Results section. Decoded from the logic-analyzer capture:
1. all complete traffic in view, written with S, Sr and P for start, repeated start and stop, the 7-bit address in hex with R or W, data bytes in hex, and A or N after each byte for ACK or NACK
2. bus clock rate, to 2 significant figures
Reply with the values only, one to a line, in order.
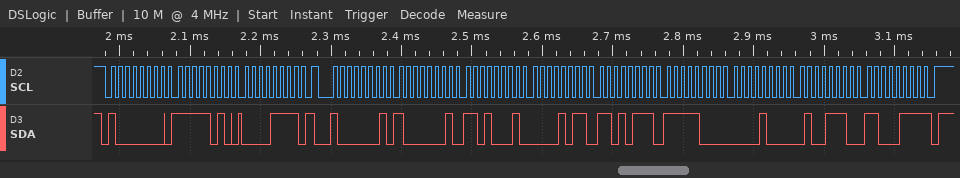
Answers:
S 40W A FA A 0F A Sr 40R A 81 A D1 A 0B A D7 A F8 A 08 A 4E A C7 N P
100 kHz
